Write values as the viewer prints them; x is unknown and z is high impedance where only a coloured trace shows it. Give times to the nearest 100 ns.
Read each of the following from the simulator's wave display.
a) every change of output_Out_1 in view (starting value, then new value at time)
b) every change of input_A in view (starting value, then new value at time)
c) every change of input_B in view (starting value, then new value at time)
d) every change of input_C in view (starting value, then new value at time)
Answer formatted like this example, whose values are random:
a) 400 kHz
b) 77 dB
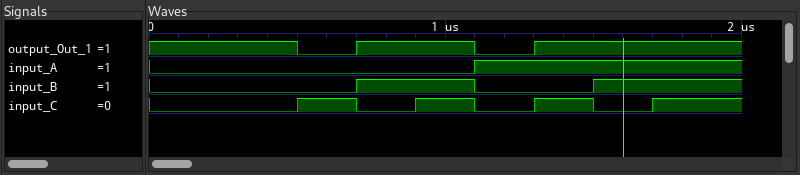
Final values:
a) 1, 0 at 500 ns, 1 at 700 ns, 0 at 1100 ns, 1 at 1300 ns
b) 0, 1 at 1100 ns
c) 0, 1 at 700 ns, 0 at 1100 ns, 1 at 1500 ns
d) 0, 1 at 500 ns, 0 at 700 ns, 1 at 900 ns, 0 at 1100 ns, 1 at 1300 ns, 0 at 1500 ns, 1 at 1700 ns
